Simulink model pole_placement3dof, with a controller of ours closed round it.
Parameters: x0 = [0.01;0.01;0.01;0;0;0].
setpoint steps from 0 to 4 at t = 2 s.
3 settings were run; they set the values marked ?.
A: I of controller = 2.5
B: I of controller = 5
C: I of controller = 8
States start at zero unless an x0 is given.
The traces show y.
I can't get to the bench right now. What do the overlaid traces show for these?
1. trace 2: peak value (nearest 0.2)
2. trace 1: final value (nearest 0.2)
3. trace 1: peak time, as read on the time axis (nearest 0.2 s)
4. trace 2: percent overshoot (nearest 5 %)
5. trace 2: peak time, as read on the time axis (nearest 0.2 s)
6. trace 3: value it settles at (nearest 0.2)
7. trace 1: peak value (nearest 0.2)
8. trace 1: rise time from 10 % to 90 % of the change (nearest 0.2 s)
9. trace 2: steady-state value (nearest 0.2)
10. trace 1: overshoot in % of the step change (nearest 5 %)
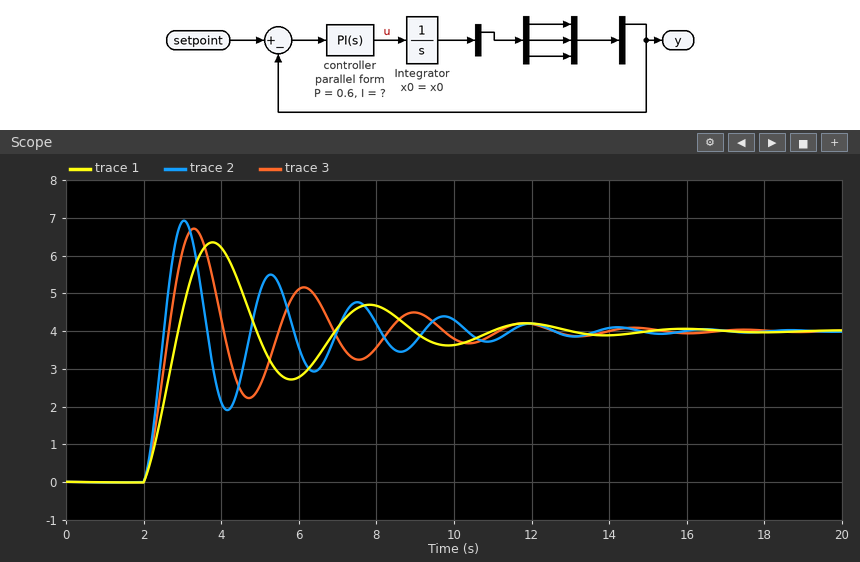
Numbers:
7.0
4.0
3.8 s
75 %
3.0 s
4.0
6.4
0.6 s
4.0
60 %
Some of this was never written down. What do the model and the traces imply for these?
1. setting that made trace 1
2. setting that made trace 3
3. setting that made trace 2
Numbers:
A
B
C
